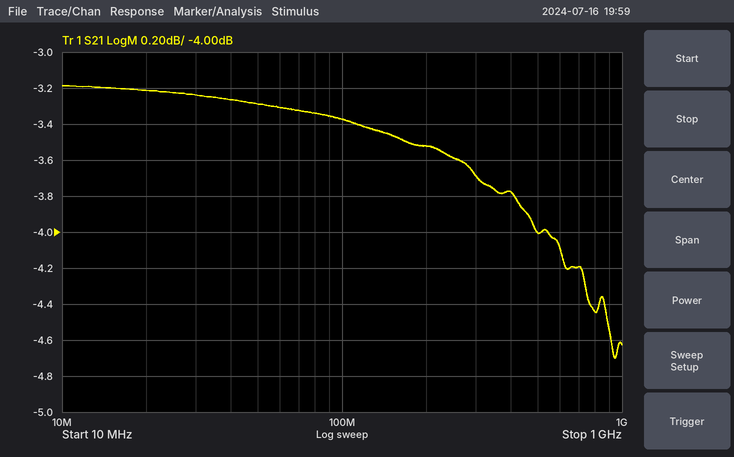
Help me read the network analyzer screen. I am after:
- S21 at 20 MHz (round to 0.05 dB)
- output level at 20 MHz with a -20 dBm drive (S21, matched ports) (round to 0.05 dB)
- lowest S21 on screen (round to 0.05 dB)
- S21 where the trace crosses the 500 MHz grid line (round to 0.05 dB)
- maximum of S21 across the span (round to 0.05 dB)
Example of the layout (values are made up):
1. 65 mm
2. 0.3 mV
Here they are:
1. -3.20 dB
2. -23.20 dBm
3. -4.70 dB
4. -4.00 dB
5. -3.20 dB
